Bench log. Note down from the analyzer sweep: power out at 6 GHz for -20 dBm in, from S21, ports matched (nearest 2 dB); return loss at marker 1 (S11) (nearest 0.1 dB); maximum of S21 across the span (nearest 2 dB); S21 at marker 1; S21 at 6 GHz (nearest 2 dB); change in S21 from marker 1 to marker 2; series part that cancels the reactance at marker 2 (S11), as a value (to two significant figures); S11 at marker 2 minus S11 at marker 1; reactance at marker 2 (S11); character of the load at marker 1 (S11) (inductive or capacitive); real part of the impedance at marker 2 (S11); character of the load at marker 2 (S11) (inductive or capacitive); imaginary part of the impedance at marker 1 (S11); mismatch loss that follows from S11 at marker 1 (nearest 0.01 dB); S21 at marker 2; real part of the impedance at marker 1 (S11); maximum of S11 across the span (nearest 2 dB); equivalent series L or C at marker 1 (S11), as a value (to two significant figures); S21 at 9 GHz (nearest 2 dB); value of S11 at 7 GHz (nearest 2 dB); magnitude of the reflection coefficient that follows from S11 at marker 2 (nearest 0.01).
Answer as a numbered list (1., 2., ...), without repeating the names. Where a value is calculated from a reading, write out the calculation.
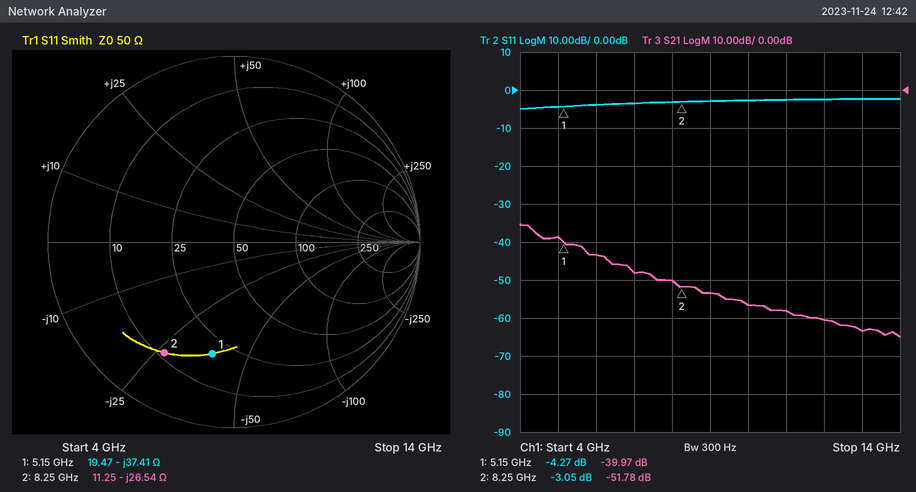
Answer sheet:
1. -20 dBm + (-44 dB) = -64 dBm
2. 4.3 dB
3. -36 dB
4. -39.97 dB
5. -44 dB
6. -51.78 − (-39.97) = -11.81 dB
7. L = 26.54 Ω/(2π × 8.25 GHz) ≈ 512 pH, so 510 pH to two significant figures
8. -3.05 − (-4.27) = 1.22 dB
9. -26.54 Ω
10. capacitive
11. 11.25 Ω
12. capacitive
13. -37.41 Ω
14. −10 log10(1 − 10^(-4.27/10)) ≈ 2.04 dB
15. -51.78 dB
16. 19.47 Ω
17. -2 dB
18. C = 1/(2π × 5.15 GHz × 37.41 Ω) ≈ 826 fF, so 830 fF to two significant figures
19. -54 dB
20. -4 dB
21. 10^(-3.05/20) ≈ 0.70
